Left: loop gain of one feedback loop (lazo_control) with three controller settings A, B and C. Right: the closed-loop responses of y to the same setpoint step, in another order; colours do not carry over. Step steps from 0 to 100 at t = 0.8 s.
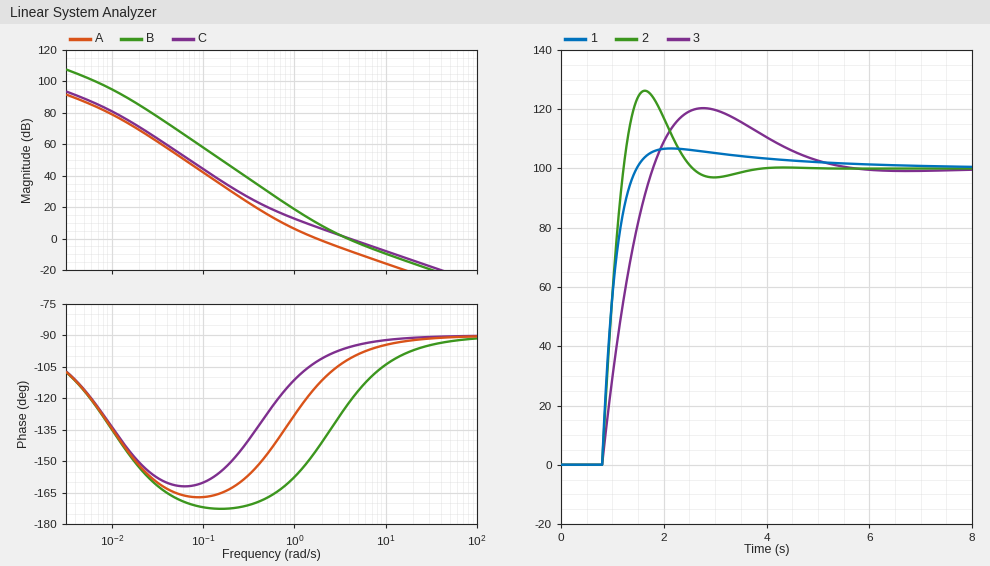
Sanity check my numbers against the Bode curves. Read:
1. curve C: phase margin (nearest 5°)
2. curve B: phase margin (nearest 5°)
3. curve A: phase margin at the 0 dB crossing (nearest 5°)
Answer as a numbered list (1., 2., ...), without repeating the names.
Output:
1. 85°
2. 55°
3. 65°
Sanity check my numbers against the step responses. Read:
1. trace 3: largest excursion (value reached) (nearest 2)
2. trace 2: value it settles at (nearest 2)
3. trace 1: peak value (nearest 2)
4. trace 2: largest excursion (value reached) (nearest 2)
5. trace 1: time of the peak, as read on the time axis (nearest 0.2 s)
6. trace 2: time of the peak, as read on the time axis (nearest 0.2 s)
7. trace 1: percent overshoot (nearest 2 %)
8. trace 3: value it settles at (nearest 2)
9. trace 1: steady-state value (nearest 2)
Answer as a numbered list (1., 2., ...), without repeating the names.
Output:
1. 120
2. 100
3. 106
4. 126
5. 2.2 s
6. 1.6 s
7. 6 %
8. 100
9. 100
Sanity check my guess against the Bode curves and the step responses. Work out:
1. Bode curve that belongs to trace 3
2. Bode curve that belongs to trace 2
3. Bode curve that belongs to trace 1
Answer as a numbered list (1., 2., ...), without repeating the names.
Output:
1. A
2. B
3. C
